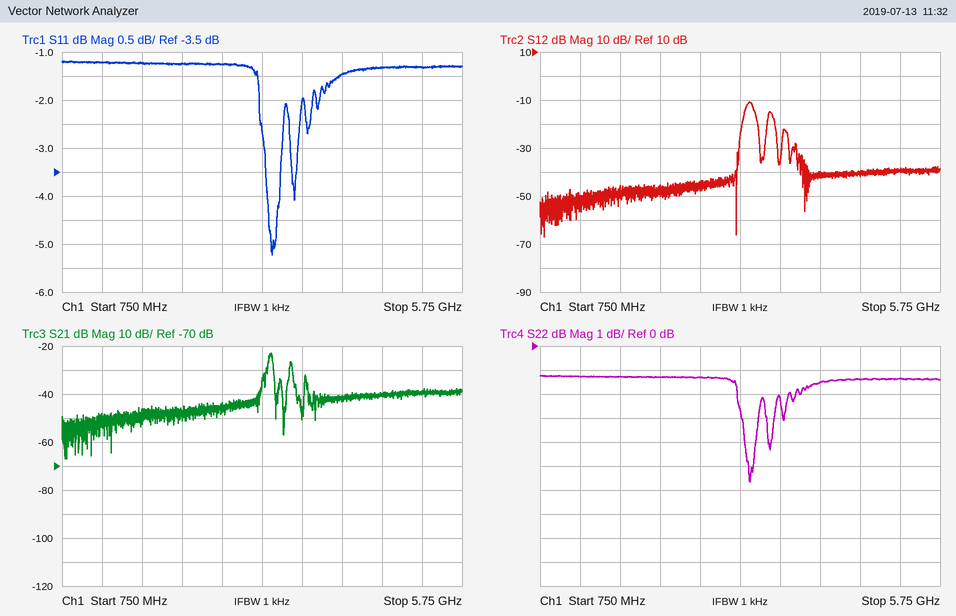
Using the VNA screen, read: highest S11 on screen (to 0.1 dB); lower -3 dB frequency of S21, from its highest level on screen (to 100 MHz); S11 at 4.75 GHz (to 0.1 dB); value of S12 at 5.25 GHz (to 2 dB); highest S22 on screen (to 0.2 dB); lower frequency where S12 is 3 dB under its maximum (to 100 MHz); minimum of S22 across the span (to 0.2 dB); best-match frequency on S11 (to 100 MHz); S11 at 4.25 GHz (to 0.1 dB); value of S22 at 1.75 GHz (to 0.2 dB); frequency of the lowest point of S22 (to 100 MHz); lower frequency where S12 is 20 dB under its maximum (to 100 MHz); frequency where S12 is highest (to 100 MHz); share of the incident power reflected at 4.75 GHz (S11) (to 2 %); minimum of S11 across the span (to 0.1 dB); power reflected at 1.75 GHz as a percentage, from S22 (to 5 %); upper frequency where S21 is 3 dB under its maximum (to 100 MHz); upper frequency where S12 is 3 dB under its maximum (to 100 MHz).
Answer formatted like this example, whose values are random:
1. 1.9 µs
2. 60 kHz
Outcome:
1. -1.2 dB
2. 3.3 GHz
3. -1.3 dB
4. -40 dB
5. -1.2 dB
6. 3.3 GHz
7. -5.6 dB
8. 3.4 GHz
9. -1.5 dB
10. -1.2 dB
11. 3.4 GHz
12. 3.2 GHz
13. 3.4 GHz
14. 74 %
15. -5.2 dB
16. 75 %
17. 3.4 GHz
18. 3.4 GHz
